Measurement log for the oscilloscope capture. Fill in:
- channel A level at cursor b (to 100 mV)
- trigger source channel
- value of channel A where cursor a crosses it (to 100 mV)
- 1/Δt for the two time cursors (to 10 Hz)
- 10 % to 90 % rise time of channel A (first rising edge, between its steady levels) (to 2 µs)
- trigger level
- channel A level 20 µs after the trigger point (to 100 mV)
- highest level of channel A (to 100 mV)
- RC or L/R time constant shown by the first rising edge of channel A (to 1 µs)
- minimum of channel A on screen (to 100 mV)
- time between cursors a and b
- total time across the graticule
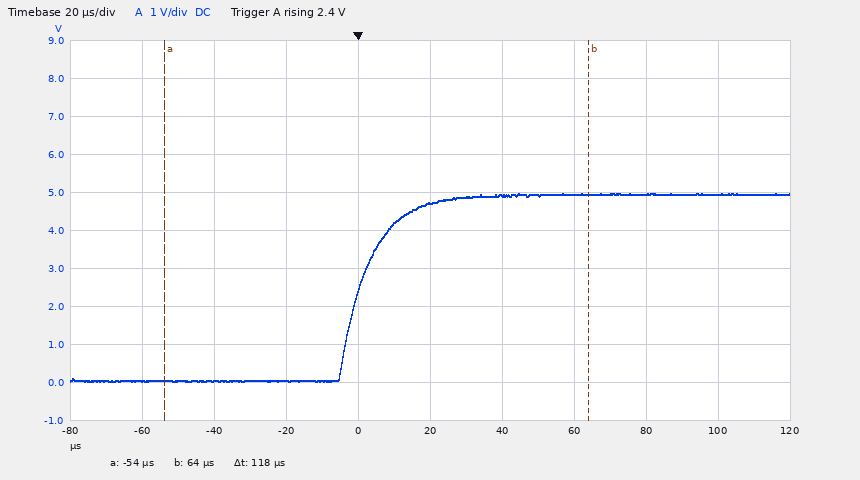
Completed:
4.9 V
channel A
100 mV
8.47 kHz
18 µs
2.4 V
4.7 V
5.0 V
8 µs
0.0 V
118 µs
200 µs
